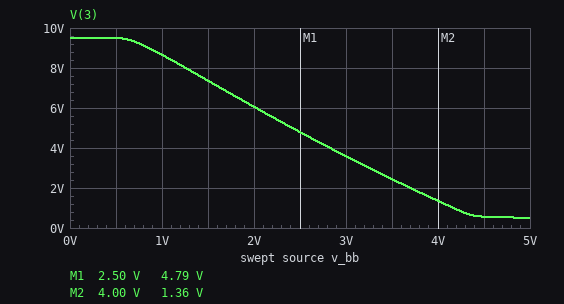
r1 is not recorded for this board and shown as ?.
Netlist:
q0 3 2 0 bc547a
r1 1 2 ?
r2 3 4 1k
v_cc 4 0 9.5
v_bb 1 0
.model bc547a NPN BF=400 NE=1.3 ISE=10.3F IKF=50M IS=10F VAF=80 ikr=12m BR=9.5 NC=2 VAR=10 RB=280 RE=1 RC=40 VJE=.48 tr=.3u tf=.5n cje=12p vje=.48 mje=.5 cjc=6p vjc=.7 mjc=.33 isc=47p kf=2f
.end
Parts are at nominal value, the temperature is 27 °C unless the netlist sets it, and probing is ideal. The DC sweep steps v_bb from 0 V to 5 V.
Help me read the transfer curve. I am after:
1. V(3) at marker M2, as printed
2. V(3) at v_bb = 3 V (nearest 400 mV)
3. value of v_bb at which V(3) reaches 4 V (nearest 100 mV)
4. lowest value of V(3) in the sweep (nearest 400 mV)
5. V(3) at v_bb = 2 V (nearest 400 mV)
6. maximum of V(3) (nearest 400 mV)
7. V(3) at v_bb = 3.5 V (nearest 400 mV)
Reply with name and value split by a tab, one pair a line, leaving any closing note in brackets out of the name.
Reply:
V(3) at marker M2, as printed	1.36 V
V(3) at v_bb = 3 V	3.6 V
value of v_bb at which V(3) reaches 4 V	2.8 V
lowest value of V(3) in the sweep	400 mV
V(3) at v_bb = 2 V	6.0 V
maximum of V(3)	9.6 V
V(3) at v_bb = 3.5 V	2.4 V
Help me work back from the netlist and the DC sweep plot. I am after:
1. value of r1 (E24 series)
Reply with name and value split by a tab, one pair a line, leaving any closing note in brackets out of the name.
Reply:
value of r1	75 kΩ
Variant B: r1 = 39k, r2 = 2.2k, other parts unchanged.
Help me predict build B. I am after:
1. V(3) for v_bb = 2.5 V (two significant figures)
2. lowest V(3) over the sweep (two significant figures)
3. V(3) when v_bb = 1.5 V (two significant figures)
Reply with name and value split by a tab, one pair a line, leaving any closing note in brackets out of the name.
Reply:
V(3) for v_bb = 2.5 V	260 mV
lowest V(3) over the sweep	230 mV
V(3) when v_bb = 1.5 V	1.1 V
